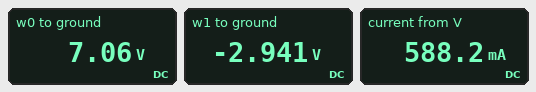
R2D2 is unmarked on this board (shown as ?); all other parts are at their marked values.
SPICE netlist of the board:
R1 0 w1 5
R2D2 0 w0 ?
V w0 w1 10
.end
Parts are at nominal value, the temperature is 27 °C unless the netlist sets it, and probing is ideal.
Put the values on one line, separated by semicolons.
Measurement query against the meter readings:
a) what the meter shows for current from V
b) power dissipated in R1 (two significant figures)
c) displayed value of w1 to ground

588.2 mA; 1.7 W; -2.941 V
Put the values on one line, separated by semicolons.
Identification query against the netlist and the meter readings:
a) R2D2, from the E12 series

12 Ω
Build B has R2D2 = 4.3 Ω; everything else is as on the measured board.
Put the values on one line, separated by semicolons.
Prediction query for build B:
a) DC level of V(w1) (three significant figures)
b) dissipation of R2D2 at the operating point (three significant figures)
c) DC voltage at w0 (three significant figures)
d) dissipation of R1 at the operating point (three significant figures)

-5.38 V; 4.97 W; 4.62 V; 5.78 W
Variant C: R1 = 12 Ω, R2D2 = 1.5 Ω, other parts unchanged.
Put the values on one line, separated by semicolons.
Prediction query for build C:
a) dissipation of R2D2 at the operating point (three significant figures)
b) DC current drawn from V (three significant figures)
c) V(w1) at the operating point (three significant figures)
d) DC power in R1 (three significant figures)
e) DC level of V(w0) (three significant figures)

823 mW; 741 mA; -8.89 V; 6.58 W; 1.11 V
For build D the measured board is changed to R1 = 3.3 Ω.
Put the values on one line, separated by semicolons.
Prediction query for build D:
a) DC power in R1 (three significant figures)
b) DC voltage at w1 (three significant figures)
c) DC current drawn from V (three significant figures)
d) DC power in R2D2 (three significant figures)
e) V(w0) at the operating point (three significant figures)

1.41 W; -2.16 V; 654 mA; 5.13 W; 7.84 V
